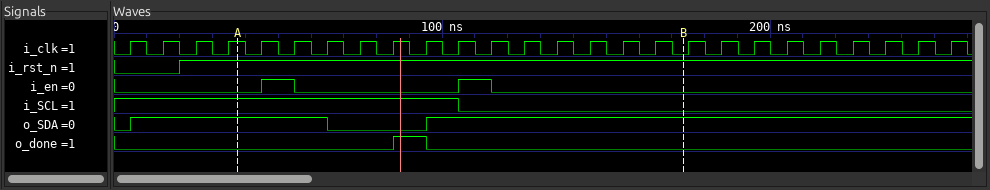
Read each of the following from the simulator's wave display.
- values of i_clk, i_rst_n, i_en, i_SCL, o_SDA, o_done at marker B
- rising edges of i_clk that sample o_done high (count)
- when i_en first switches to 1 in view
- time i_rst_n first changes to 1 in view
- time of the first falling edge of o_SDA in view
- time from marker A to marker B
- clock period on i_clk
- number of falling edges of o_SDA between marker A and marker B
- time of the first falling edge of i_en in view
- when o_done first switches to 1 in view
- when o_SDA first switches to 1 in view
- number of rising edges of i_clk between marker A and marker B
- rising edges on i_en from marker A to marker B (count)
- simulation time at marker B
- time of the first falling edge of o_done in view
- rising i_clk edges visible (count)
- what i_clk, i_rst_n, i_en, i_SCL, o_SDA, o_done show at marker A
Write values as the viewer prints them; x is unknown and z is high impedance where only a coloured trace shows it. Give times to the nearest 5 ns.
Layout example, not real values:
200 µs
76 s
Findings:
i_clk=0, i_rst_n=1, i_en=0, i_SCL=0, o_SDA=1, o_done=0
1
45 ns
20 ns
65 ns
135 ns
10 ns
1
55 ns
85 ns
5 ns
13
2
175 ns
95 ns
26
i_clk=1, i_rst_n=1, i_en=0, i_SCL=1, o_SDA=1, o_done=0
